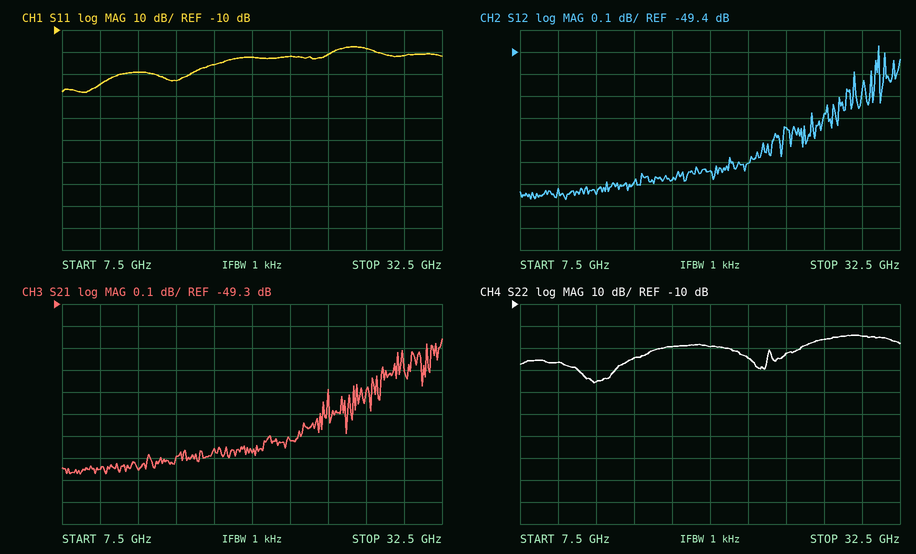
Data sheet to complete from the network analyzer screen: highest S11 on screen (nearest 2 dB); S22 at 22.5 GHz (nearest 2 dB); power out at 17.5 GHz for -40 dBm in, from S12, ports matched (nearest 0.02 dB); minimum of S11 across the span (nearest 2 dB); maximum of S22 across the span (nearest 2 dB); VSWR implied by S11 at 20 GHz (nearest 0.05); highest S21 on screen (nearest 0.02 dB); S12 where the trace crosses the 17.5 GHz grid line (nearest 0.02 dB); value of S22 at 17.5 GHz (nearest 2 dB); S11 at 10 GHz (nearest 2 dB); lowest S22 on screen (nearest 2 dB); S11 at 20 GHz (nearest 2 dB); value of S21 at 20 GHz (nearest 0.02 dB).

-18 dB
-34 dB
-89.98 dBm
-38 dB
-24 dB
1.15
-49.46 dB
-49.98 dB
-30 dB
-34 dB
-46 dB
-22 dB
-49.98 dB
